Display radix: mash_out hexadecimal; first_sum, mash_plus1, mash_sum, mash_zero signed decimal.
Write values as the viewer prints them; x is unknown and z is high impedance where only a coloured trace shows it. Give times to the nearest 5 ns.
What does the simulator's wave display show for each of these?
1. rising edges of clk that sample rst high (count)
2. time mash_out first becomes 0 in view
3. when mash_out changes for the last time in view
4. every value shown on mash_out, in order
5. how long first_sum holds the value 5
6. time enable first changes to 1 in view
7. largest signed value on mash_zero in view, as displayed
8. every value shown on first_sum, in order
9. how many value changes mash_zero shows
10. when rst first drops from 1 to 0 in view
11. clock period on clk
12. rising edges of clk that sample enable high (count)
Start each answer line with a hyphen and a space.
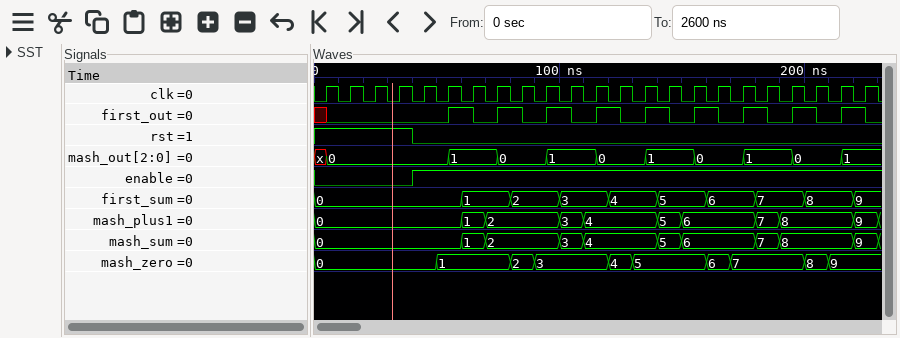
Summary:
- 4
- 5 ns
- 215 ns
- x, 0, 1, 0, 1, 0, 1, 0, 1, 0, 1
- 20 ns
- 40 ns
- 9
- 0, 1, 2, 3, 4, 5, 6, 7, 8, 9
- 9
- 40 ns
- 10 ns
- 19
